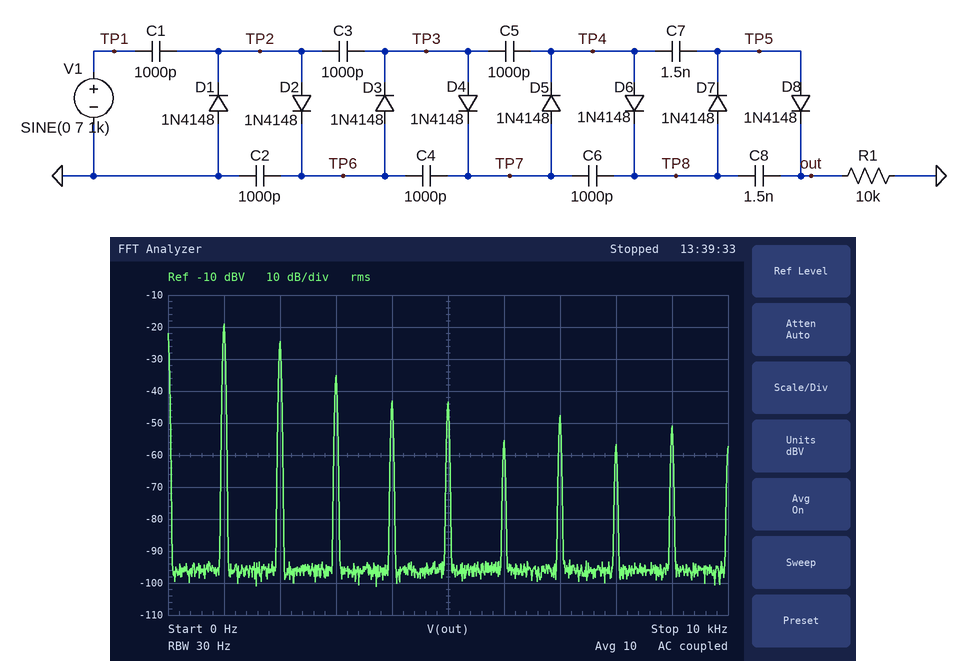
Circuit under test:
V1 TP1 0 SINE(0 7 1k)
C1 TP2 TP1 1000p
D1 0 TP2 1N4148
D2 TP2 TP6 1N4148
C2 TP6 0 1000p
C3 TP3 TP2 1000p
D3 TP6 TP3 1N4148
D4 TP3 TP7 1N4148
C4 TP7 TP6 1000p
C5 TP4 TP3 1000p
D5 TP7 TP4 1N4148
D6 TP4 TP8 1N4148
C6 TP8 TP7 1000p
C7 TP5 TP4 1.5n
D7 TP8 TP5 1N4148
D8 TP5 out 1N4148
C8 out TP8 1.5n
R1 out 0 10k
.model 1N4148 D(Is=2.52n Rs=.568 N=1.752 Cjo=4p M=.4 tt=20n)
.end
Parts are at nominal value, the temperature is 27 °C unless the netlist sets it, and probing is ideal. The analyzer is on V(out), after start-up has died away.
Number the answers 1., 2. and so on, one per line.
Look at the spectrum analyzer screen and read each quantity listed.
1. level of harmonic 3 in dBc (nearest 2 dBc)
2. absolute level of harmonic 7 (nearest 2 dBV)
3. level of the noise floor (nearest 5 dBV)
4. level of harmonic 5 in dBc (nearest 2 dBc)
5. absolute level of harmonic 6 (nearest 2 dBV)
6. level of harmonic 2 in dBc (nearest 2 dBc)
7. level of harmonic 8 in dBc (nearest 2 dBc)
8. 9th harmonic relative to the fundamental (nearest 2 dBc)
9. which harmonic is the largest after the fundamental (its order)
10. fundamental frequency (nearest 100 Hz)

1. -16 dBc
2. -48 dBV
3. -95 dBV
4. -24 dBc
5. -56 dBV
6. -6 dBc
7. -38 dBc
8. -32 dBc
9. 2
10. 1.0 kHz
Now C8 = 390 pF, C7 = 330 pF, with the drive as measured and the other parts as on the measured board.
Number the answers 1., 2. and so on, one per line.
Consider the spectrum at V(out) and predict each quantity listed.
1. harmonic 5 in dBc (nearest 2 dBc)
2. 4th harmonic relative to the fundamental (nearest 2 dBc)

1. -28 dBc
2. -30 dBc
